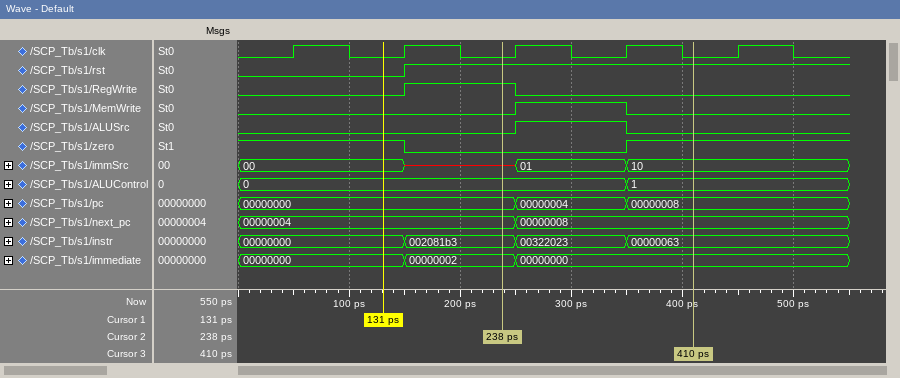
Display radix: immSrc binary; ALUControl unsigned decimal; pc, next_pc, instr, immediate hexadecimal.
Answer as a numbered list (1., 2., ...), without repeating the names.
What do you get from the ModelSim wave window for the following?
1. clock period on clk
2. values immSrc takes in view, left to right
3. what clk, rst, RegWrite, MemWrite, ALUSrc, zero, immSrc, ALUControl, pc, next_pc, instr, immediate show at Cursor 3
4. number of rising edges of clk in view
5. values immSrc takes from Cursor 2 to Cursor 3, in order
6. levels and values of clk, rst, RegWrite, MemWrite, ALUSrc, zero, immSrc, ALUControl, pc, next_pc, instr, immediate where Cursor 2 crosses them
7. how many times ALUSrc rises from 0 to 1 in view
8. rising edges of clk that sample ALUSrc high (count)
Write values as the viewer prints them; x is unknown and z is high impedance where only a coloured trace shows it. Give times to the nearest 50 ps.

1. 100 ps
2. 00, x, 01, 10
3. clk=0, rst=1, RegWrite=0, MemWrite=0, ALUSrc=0, zero=1, immSrc=10, ALUControl=1, pc=00000008, next_pc=00000008, instr=00000063, immediate=00000000
4. 5
5. x, 01, 10
6. clk=0, rst=1, RegWrite=1, MemWrite=0, ALUSrc=0, zero=0, immSrc=x, ALUControl=0, pc=00000000, next_pc=00000004, instr=002081b3, immediate=00000002
7. 1
8. 1
